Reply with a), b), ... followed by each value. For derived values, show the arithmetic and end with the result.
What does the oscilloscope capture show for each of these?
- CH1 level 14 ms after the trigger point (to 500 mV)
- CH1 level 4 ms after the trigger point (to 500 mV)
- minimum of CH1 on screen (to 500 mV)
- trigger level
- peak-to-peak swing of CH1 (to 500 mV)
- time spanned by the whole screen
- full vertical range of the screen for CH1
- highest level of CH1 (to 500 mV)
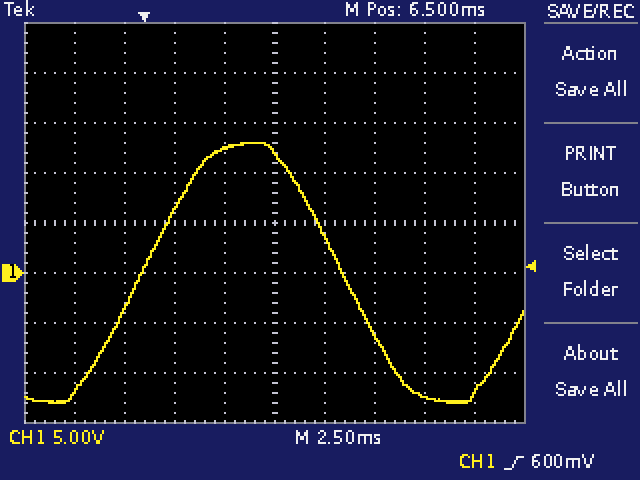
a) -12.5 V
b) 12.5 V
c) -13.0 V
d) 600 mV
e) 13.0 V − (-13.0 V) = 26.0 V
f) 25 ms
g) 40 V
h) 13.0 V
